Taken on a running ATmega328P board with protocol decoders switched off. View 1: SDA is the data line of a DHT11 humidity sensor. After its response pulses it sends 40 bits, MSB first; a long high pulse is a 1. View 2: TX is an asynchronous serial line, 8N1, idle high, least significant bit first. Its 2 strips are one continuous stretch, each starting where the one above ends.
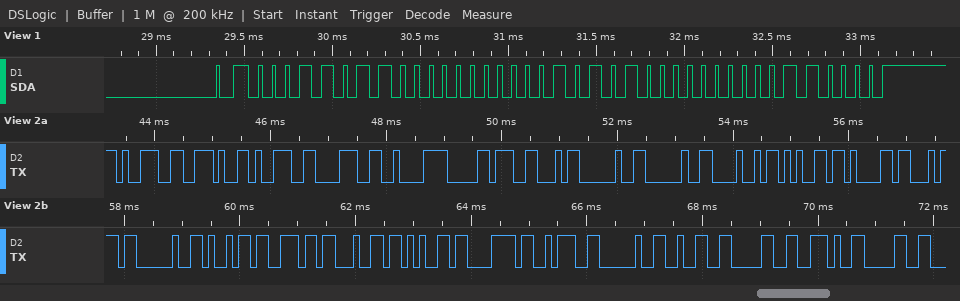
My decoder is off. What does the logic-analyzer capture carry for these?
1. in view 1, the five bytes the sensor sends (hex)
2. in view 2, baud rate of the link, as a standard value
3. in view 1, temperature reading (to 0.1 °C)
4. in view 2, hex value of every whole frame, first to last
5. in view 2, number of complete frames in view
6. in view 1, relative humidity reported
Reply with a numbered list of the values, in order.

1. 1B 00 15 00 30
2. 9600 baud
3. 21.0 °C
4. 0x39 0x2E 0x39 0x38 0xC2 0xB0 0x46 0x20 0x20 0x48 0x65 0x61 0x74 0x20 0x69 0x6E 0x64 0x65 0x78 0x3A 0x20 0x32 0x30 0x2E 0x30
5. 25
6. 27 %
